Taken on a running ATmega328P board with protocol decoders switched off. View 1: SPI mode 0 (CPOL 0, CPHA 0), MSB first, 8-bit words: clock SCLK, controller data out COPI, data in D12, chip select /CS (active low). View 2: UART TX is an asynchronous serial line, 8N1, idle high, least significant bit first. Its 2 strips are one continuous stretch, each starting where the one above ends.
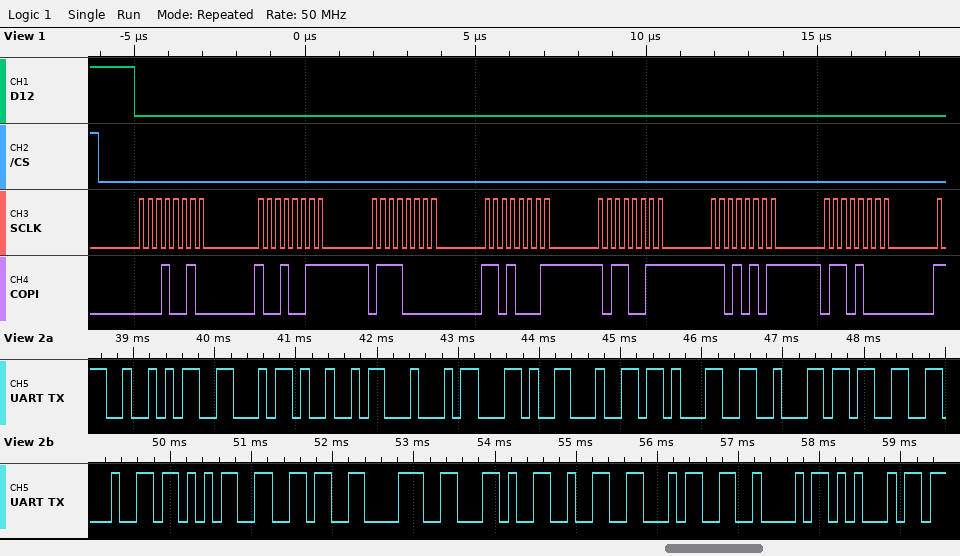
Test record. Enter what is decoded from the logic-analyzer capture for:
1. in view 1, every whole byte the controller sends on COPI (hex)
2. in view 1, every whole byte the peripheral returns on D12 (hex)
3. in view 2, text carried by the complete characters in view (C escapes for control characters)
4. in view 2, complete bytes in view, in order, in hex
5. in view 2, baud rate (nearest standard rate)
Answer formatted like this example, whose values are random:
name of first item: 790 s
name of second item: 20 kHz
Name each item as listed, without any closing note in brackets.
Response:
in view 1, every whole byte the controller sends on COPI: 12 93 70 D1 B3 D5 68
in view 1, every whole byte the peripheral returns on D12: 00 00 00 00 00 00 00
in view 2, text carried by the complete characters in view: "RFID,d1b3d568,24BE"
in view 2, complete bytes in view, in order, in hex: 52 46 49 44 2C 64 31 62 33 64 35 36 38 2C 32 34 42 45
in view 2, baud rate: 9600 baud
